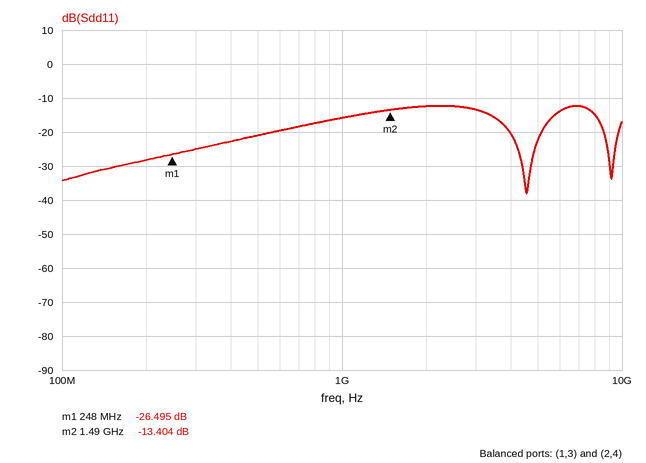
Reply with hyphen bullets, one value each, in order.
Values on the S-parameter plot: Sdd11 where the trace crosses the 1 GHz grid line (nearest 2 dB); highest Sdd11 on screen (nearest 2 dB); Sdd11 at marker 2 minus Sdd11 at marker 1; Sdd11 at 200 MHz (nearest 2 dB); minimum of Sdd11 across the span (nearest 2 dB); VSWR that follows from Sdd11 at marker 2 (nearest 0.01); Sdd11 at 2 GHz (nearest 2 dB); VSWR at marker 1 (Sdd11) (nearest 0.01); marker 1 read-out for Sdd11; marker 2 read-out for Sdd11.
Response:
- -16 dB
- -12 dB
- 13.091 dB
- -28 dB
- -38 dB
- 1.54
- -12 dB
- 1.10
- -26.495 dB
- -13.404 dB
